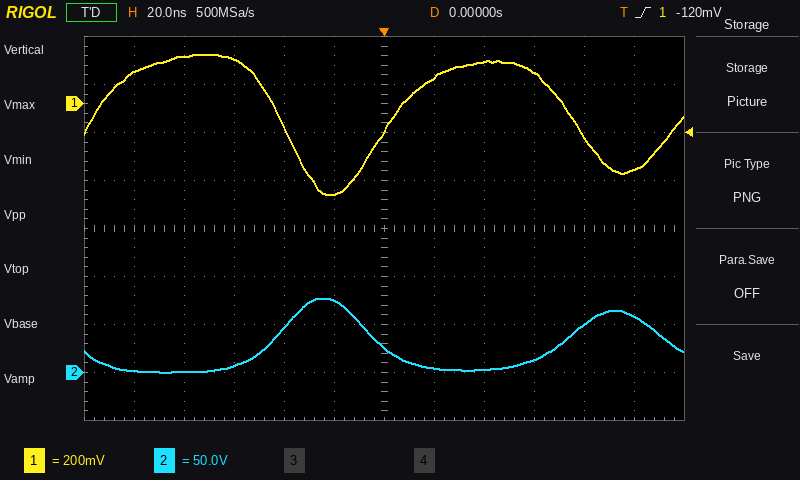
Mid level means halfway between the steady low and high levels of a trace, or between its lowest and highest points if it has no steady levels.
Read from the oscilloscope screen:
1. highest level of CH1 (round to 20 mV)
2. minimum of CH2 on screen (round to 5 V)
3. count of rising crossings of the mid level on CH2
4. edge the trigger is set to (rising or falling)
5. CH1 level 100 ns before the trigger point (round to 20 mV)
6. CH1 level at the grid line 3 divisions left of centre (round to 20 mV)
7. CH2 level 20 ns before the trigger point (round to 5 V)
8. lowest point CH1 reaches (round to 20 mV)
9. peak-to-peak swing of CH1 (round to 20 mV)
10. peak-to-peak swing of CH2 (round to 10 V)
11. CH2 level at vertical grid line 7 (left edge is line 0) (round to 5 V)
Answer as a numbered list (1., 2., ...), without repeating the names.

1. 200 mV
2. 0 V
3. 2
4. rising
5. 140 mV
6. 180 mV
7. 75 V
8. -380 mV
9. 580 mV
10. 80 V
11. 5 V
